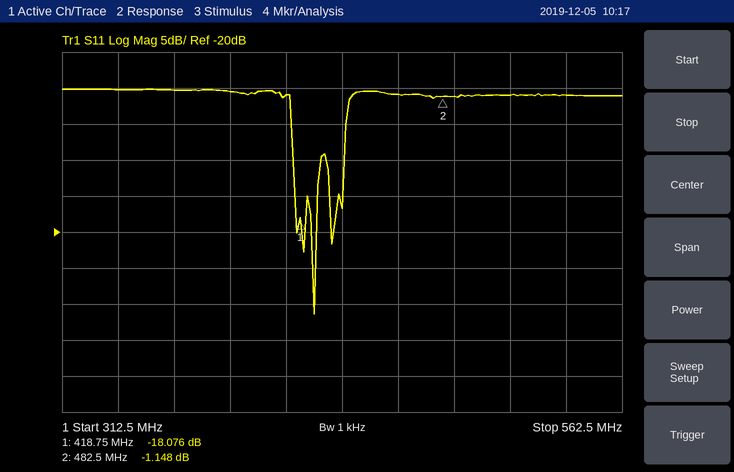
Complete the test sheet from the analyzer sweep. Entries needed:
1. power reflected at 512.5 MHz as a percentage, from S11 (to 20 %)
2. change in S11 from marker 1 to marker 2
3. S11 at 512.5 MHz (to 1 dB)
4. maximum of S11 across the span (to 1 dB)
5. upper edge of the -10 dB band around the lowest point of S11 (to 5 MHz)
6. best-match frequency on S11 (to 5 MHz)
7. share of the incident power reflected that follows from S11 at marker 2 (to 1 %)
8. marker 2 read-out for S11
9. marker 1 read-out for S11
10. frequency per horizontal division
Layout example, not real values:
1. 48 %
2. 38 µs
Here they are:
1. 80 %
2. 16.928 dB
3. -1 dB
4. 0 dB
5. 430 MHz
6. 425 MHz
7. 77 %
8. -1.148 dB
9. -18.076 dB
10. 25 MHz
